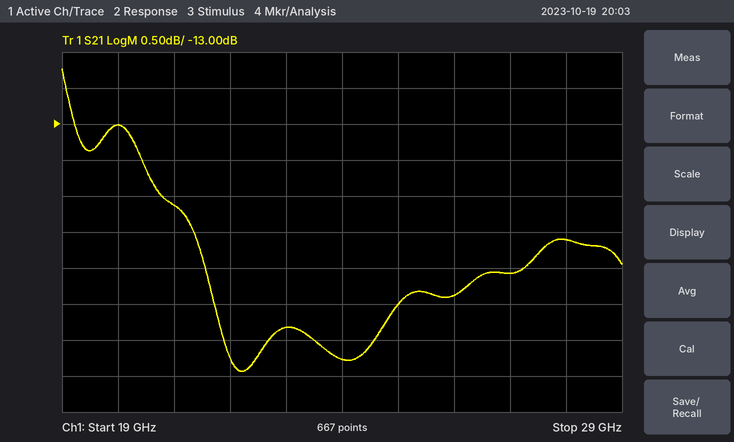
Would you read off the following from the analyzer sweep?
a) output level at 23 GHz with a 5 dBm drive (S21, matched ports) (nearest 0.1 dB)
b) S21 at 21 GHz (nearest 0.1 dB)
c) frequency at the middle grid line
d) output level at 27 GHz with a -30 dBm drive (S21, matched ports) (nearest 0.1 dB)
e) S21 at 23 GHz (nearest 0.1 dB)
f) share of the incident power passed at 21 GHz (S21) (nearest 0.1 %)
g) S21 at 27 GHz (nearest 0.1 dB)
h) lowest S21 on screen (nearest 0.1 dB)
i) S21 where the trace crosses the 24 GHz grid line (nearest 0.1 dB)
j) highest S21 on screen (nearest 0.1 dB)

-10.8 dBm
-14.1 dB
24 GHz
-45.1 dBm
-15.8 dB
3.9 %
-15.1 dB
-16.4 dB
-16.3 dB
-12.2 dB
